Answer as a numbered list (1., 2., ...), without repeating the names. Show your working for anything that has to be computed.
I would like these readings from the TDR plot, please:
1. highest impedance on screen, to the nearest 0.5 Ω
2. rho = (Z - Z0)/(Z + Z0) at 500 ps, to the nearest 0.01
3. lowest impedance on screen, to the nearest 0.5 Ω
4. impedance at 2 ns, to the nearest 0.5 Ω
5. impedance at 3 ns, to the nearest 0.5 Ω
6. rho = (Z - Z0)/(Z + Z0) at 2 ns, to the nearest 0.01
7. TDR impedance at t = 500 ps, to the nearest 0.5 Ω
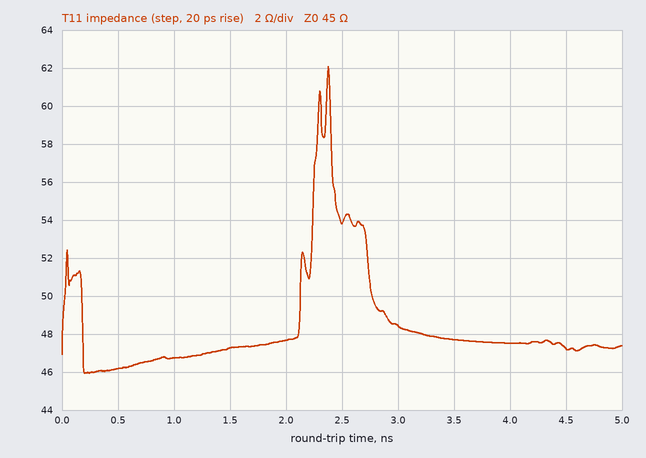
1. 62.0 Ω
2. (46 − 45)/(46 + 45) ≈ +0.01
3. 46.0 Ω
4. 47.5 Ω
5. 48.5 Ω
6. (47.5 − 45)/(47.5 + 45) ≈ +0.03
7. 46.0 Ω
